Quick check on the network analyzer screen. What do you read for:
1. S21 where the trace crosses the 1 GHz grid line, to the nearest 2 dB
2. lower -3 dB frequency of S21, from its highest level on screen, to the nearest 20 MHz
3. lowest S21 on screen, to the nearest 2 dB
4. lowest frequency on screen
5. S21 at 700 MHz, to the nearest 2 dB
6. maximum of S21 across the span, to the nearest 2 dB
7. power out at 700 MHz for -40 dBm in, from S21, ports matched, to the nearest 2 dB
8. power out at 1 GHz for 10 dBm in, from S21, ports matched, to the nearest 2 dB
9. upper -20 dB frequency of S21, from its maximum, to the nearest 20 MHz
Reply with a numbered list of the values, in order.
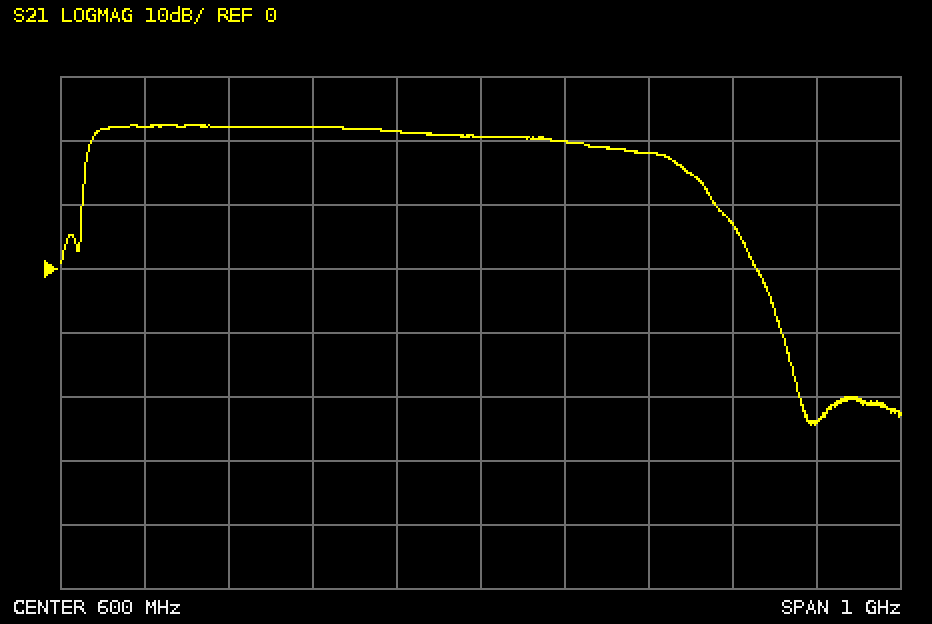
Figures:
1. -24 dB
2. 140 MHz
3. -24 dB
4. 100 MHz
5. 20 dB
6. 22 dB
7. -20 dBm
8. -14 dBm
9. 920 MHz
